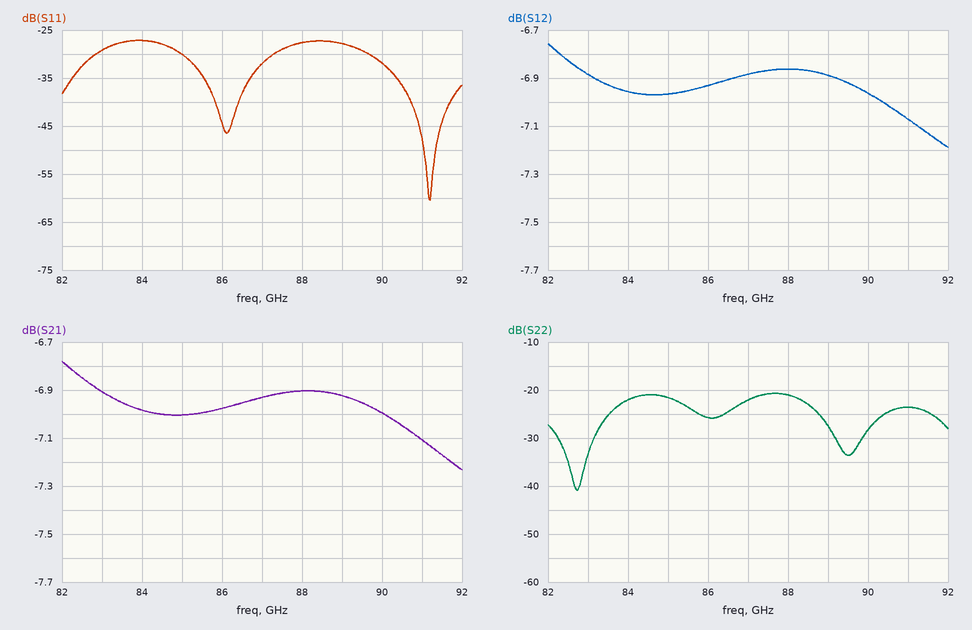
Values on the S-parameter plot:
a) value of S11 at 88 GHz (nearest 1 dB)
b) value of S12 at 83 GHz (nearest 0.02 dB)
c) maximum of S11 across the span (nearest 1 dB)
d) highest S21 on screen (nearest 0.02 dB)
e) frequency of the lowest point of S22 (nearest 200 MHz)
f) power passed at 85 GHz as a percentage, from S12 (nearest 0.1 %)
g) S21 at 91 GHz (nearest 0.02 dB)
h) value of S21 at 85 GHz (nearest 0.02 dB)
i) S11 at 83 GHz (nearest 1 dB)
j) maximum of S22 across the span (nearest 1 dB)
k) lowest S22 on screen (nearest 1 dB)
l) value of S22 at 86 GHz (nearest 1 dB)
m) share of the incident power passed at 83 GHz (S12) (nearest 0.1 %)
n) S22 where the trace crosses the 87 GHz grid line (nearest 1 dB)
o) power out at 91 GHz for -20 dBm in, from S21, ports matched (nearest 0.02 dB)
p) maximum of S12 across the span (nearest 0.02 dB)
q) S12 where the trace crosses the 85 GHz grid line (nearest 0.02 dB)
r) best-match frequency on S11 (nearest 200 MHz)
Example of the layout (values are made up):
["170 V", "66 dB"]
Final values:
["-28 dB", "-6.88 dB", "-27 dB", "-6.78 dB", "82.8 GHz", "20.1 %", "-7.10 dB", "-7.00 dB", "-29 dB", "-21 dB", "-41 dB", "-26 dB", "20.5 %", "-22 dB", "-27.10 dBm", "-6.76 dB", "-6.96 dB", "91.2 GHz"]
